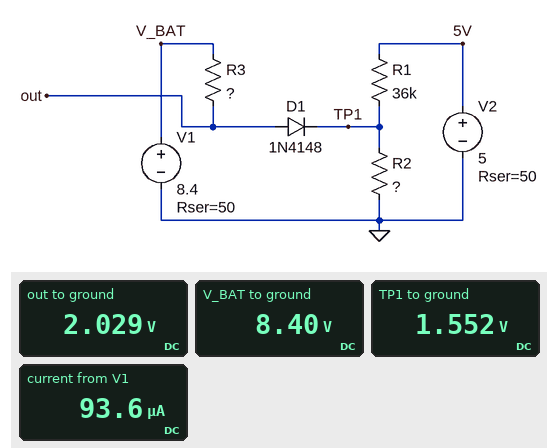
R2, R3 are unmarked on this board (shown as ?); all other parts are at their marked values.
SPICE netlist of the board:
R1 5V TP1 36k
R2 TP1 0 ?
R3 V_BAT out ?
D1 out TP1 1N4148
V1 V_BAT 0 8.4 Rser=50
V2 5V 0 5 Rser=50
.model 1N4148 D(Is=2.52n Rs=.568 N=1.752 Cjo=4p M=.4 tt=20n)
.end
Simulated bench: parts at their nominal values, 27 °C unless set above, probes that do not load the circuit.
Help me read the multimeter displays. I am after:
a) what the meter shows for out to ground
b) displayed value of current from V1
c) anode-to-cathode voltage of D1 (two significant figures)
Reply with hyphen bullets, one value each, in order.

- 2.029 V
- 93.6 µA
- 480 mV
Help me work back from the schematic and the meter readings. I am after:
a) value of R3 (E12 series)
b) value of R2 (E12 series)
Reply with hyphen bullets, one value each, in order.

- 68 kΩ
- 8.2 kΩ
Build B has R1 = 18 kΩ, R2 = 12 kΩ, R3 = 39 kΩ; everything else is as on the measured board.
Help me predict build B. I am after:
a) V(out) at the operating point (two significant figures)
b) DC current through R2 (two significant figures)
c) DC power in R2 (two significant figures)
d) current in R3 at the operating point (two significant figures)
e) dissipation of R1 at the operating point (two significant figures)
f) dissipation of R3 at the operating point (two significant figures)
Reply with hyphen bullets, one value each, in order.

- 3.4 V
- 240 µA
- 710 µW
- 130 µA
- 240 µW
- 640 µW
